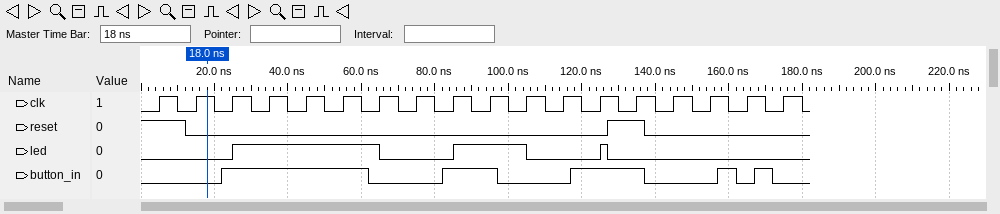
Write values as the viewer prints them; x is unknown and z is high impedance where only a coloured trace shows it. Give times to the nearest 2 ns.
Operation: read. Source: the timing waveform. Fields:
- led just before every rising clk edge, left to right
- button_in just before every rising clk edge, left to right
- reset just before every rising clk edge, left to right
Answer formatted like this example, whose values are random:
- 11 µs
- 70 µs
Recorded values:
- 0 0 0 1 1 1 1 0 0 1 1 0 0 0 0 0 0 0
- 0 0 1 1 1 1 0 0 1 1 0 0 1 1 0 0 0 0
- 1 0 0 0 0 0 0 0 0 0 0 0 0 1 0 0 0 0
